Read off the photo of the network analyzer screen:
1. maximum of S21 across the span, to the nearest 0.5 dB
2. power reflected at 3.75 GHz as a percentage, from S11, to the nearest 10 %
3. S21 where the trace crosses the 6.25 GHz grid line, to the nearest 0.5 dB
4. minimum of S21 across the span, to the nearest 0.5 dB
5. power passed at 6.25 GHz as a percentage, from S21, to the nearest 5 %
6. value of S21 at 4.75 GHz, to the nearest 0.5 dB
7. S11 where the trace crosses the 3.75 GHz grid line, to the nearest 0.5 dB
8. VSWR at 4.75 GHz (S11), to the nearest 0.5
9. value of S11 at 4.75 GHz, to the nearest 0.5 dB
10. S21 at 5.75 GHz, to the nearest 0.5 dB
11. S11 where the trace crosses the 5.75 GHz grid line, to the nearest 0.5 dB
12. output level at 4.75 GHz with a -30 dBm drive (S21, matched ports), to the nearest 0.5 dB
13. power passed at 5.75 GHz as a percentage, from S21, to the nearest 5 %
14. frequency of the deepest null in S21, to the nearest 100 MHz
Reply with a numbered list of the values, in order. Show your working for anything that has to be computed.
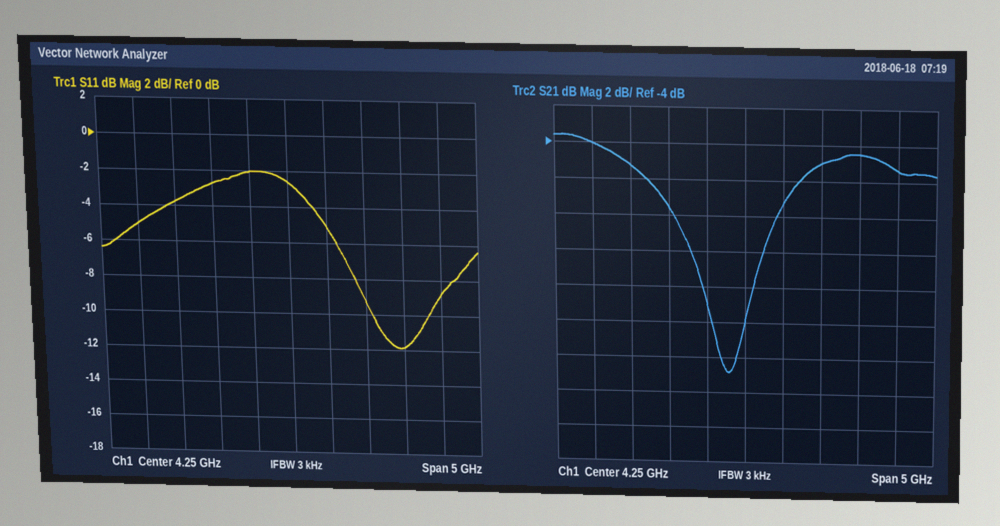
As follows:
1. -3.5 dB
2. 10^(-2/10) ≈ 63.1 %, so 60 % to the nearest 10 %
3. -5.5 dB
4. -17.0 dB
5. 10^(-5.5/10) ≈ 28.2 %, so 30 % to the nearest 5 %
6. -7.5 dB
7. -2.0 dB
8. |Γ| = 10^(-5/20) = 0.5623; VSWR = (1 + 0.5623)/(1 − 0.5623) ≈ 3.57, so 3.5 to the nearest 0.5
9. -5.0 dB
10. -4.5 dB
11. -12.0 dB
12. -30 dBm + (-7.5 dB) = -37.5 dBm
13. 10^(-4.5/10) ≈ 35 %
14. 4.0 GHz
